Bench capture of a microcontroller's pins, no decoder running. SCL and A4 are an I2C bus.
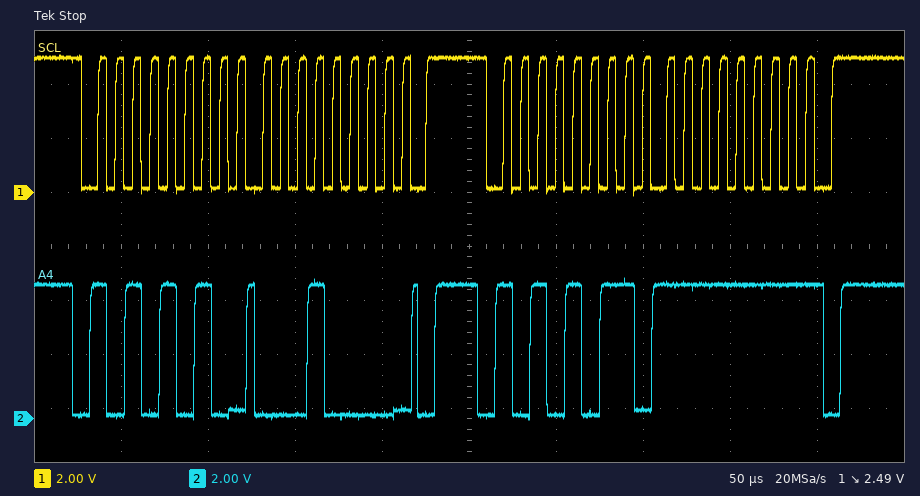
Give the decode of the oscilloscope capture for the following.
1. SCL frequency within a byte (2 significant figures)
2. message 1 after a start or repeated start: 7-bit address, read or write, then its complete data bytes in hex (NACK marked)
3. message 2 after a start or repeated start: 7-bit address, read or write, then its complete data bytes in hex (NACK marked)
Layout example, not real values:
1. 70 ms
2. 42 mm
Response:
1. 100 kHz
2. 0x55 write: 10
3. 0x55 read: FF NACK
